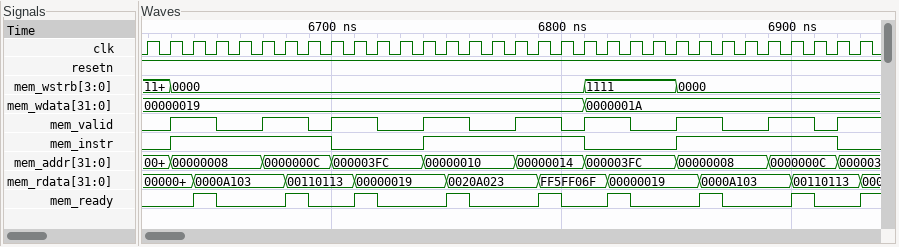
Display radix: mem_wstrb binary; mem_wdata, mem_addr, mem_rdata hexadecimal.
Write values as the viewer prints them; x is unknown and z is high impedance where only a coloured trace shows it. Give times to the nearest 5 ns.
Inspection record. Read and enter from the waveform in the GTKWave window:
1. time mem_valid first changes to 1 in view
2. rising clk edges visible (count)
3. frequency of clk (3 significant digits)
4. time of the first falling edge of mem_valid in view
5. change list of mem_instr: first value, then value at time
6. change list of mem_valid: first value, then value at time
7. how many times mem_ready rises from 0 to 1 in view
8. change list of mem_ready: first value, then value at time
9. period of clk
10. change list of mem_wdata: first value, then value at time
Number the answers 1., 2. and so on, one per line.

1. 6630 ns
2. 32
3. 100 MHz
4. 6650 ns
5. 0, 1 at 6630 ns, 0 at 6700 ns, 1 at 6740 ns, 0 at 6810 ns, 1 at 6850 ns, 0 at 6920 ns
6. 0, 1 at 6630 ns, 0 at 6650 ns, 1 at 6670 ns, 0 at 6690 ns, 1 at 6700 ns, 0 at 6720 ns, 1 at 6740 ns, 0 at 6760 ns, 1 at 6780 ns, 0 at 6800 ns, 1 at 6810 ns, 0 at 6830 ns, 1 at 6850 ns, 0 at 6870 ns, 1 at 6890 ns, 0 at 6910 ns, 1 at 6920 ns
7. 9
8. 0, 1 at 6640 ns, 0 at 6650 ns, 1 at 6680 ns, 0 at 6690 ns, 1 at 6710 ns, 0 at 6720 ns, 1 at 6750 ns, 0 at 6760 ns, 1 at 6790 ns, 0 at 6800 ns, 1 at 6820 ns, 0 at 6830 ns, 1 at 6860 ns, 0 at 6870 ns, 1 at 6900 ns, 0 at 6910 ns, 1 at 6930 ns
9. 10 ns
10. 00000019, 0000001A at 6810 ns
